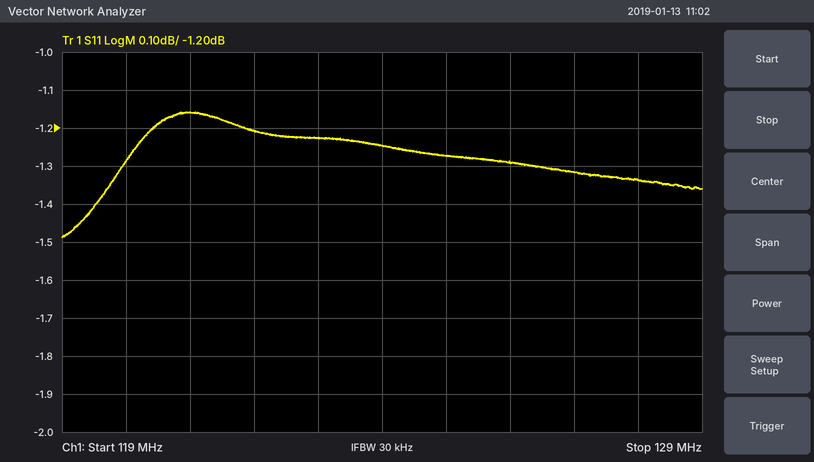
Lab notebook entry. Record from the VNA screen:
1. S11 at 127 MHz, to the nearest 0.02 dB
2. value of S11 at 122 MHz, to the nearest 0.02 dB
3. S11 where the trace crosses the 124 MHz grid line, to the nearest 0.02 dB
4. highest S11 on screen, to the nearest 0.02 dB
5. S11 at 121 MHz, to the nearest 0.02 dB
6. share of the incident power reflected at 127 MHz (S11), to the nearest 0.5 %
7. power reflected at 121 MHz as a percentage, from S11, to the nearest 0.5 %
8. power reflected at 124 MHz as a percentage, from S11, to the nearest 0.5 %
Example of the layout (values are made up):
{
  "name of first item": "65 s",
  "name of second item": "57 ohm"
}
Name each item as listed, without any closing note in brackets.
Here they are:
{
  "S11 at 127 MHz, to the nearest 0.02 dB": "-1.32 dB",
  "value of S11 at 122 MHz, to the nearest 0.02 dB": "-1.20 dB",
  "S11 where the trace crosses the 124 MHz grid line, to the nearest 0.02 dB": "-1.24 dB",
  "highest S11 on screen, to the nearest 0.02 dB": "-1.16 dB",
  "S11 at 121 MHz, to the nearest 0.02 dB": "-1.16 dB",
  "share of the incident power reflected at 127 MHz (S11), to the nearest 0.5 %": "74.0 %",
  "power reflected at 121 MHz as a percentage, from S11, to the nearest 0.5 %": "76.5 %",
  "power reflected at 124 MHz as a percentage, from S11, to the nearest 0.5 %": "75.0 %"
}
